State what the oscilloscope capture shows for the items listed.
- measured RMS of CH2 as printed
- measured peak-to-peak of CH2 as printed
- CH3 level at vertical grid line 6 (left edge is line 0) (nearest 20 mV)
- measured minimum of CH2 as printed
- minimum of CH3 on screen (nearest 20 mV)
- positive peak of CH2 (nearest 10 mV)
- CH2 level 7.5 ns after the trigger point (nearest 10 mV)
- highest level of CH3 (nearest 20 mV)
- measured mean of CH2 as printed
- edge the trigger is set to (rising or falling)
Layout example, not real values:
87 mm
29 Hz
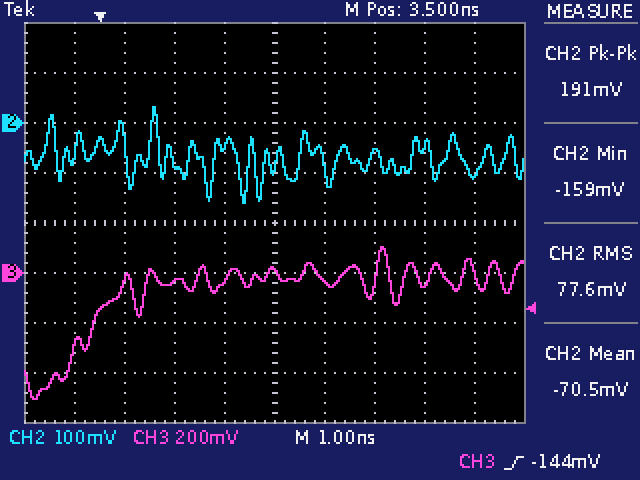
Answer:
77.6 mV
191 mV
-40 mV
-159 mV
-500 mV
30 mV
-100 mV
100 mV
-70.5 mV
rising
